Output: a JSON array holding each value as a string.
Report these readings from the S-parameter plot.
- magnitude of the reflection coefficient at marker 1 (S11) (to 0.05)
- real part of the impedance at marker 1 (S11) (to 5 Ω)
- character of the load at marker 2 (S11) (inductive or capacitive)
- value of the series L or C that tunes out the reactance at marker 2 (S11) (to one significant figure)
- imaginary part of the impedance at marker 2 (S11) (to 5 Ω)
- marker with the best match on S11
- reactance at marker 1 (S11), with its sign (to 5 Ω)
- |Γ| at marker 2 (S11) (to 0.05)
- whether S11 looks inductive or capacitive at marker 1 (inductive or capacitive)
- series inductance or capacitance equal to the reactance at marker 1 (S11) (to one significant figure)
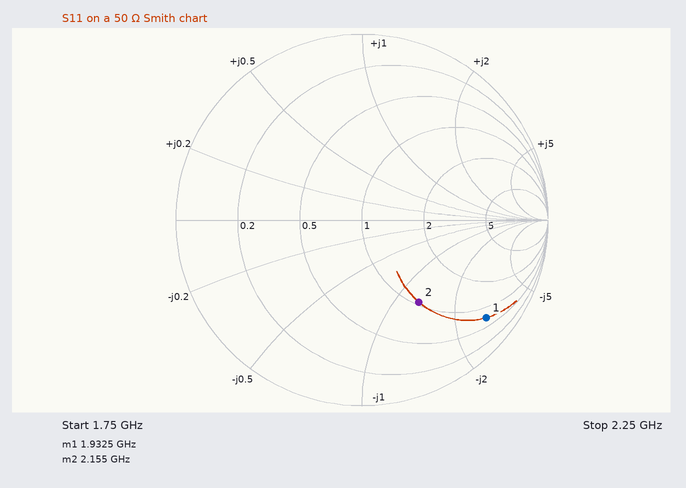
["0.85", "35 Ω", "capacitive", "5 nH", "-65 Ω", "marker 2", "-135 Ω", "0.55", "capacitive", "600 fF"]
